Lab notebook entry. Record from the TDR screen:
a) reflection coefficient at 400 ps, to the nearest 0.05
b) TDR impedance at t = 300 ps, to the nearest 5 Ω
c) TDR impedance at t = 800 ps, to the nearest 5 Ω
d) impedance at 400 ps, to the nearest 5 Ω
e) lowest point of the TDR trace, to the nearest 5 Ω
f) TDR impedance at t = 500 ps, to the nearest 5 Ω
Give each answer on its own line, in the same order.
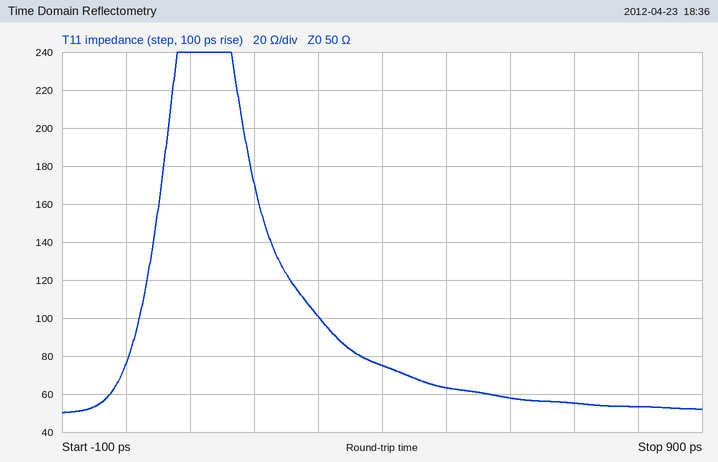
+0.20
100 Ω
55 Ω
75 Ω
50 Ω
65 Ω
